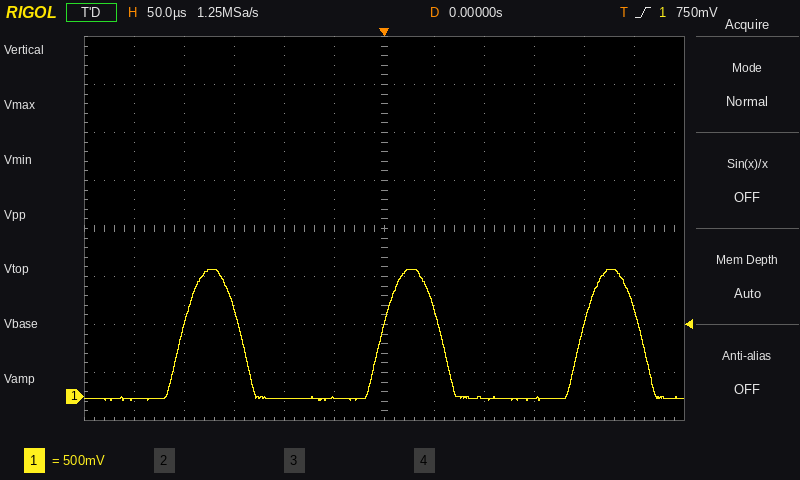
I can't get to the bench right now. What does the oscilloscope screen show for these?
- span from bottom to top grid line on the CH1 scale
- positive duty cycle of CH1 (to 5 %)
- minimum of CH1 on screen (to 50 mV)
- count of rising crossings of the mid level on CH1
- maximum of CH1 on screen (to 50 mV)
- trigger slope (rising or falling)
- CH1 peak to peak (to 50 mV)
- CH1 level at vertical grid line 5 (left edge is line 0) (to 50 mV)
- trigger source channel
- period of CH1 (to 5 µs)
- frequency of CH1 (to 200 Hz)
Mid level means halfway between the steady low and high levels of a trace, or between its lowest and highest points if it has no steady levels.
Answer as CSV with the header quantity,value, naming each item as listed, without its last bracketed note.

quantity,value
span from bottom to top grid line on the CH1 scale,4 V
positive duty cycle of CH1,30 %
minimum of CH1 on screen,-50 mV
count of rising crossings of the mid level on CH1,3
maximum of CH1 on screen,1.30 V
trigger slope,rising
CH1 peak to peak,1.35 V
CH1 level at vertical grid line 5 (left edge is line 0),0 mV
trigger source channel,CH1
period of CH1,200 µs
frequency of CH1,5.0 kHz
